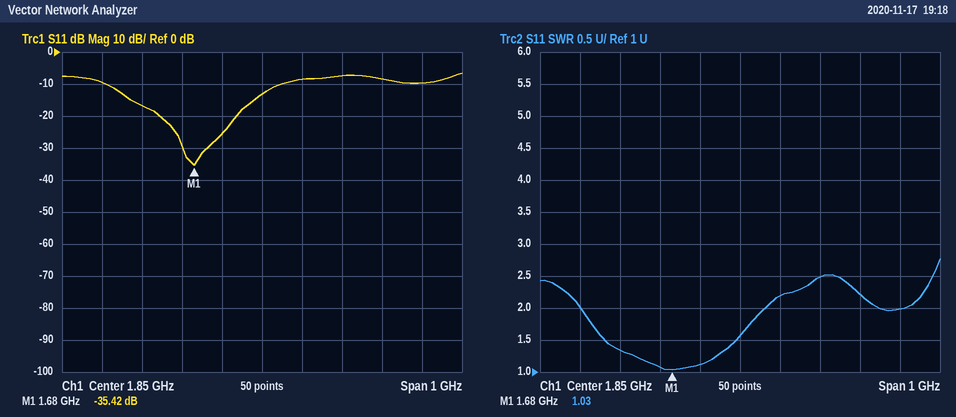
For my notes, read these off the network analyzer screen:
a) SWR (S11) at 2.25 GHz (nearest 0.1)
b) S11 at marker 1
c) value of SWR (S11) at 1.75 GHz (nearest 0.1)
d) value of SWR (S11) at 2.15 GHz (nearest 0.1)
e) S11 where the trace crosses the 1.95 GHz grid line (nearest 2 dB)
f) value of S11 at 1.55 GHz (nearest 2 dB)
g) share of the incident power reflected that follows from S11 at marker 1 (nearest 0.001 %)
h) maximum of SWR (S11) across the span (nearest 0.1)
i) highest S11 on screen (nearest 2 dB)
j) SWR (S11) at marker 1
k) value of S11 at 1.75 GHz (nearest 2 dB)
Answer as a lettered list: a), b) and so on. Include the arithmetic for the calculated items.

a) 2.0
b) -35.42 dB
c) 1.1
d) 2.2
e) -8 dB
f) -16 dB
g) 10^(-35.42/10) ≈ 0.029 %
h) 2.8
i) -6 dB
j) 1.03
k) -26 dB
